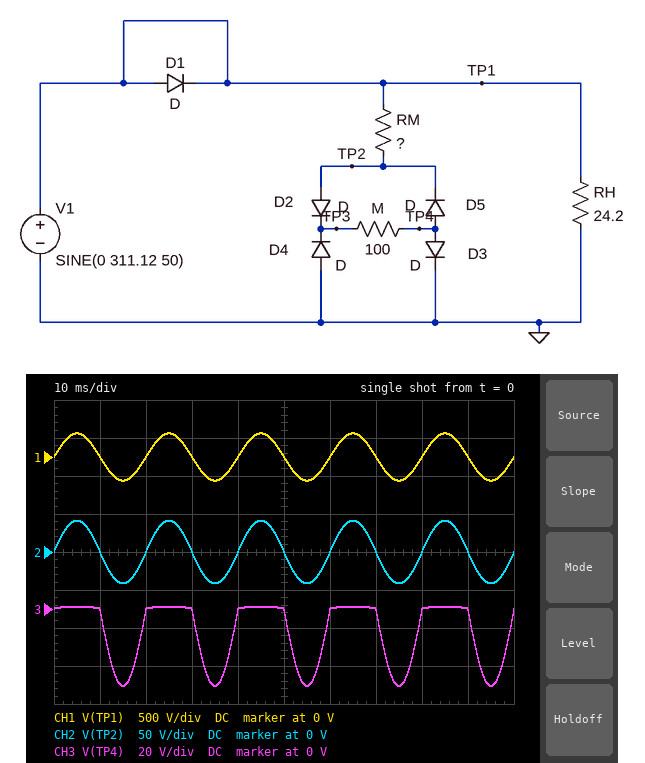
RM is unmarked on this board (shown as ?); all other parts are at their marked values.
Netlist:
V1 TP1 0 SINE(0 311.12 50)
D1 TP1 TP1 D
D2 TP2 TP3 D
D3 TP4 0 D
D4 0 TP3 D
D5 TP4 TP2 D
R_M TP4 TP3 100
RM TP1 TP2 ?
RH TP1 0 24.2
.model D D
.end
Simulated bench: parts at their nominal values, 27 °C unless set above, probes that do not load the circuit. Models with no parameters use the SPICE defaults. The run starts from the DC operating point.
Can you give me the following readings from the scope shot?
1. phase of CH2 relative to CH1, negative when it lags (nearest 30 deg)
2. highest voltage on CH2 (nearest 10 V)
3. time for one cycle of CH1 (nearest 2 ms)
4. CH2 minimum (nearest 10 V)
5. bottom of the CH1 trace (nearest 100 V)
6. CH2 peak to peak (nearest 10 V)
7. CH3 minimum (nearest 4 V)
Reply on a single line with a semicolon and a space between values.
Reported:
0 deg; 40 V; 20 ms; -40 V; -300 V; 80 V; -40 V
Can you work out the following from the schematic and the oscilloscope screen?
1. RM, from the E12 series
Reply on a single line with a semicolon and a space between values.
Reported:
680 Ω
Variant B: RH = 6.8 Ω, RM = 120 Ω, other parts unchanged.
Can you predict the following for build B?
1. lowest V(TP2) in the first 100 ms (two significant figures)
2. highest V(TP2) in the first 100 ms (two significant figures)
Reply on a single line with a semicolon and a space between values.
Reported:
-140 V; 140 V
